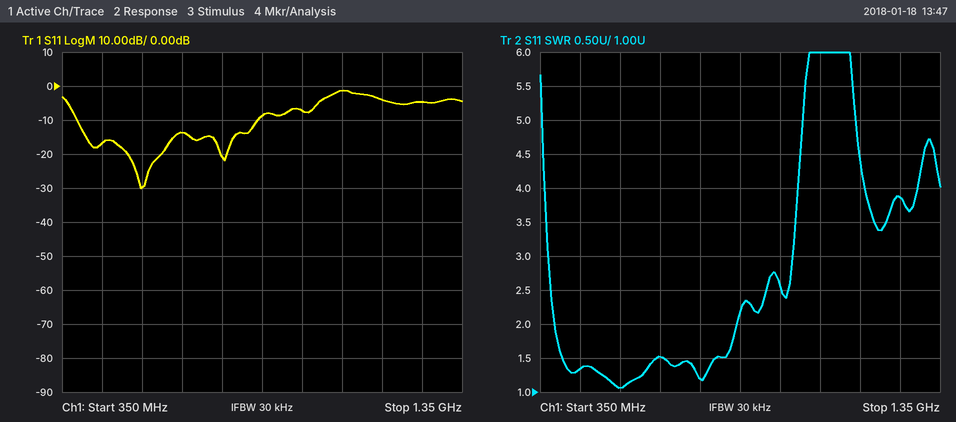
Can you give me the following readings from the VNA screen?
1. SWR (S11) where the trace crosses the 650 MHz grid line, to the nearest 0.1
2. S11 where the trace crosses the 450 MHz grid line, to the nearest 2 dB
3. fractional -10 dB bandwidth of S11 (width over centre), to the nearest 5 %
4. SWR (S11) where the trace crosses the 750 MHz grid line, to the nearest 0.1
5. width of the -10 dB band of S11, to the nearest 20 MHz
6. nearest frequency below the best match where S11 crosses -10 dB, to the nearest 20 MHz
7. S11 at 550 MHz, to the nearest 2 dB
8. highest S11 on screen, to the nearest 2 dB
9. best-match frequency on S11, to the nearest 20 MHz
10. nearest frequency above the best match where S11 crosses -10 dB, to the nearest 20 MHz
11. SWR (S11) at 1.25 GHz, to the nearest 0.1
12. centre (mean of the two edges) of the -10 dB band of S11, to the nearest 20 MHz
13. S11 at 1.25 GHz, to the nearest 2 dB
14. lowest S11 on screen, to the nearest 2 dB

1.5
-16 dB
75 %
1.2
460 MHz
380 MHz
-30 dB
-2 dB
540 MHz
840 MHz
3.9
620 MHz
-4 dB
-30 dB
